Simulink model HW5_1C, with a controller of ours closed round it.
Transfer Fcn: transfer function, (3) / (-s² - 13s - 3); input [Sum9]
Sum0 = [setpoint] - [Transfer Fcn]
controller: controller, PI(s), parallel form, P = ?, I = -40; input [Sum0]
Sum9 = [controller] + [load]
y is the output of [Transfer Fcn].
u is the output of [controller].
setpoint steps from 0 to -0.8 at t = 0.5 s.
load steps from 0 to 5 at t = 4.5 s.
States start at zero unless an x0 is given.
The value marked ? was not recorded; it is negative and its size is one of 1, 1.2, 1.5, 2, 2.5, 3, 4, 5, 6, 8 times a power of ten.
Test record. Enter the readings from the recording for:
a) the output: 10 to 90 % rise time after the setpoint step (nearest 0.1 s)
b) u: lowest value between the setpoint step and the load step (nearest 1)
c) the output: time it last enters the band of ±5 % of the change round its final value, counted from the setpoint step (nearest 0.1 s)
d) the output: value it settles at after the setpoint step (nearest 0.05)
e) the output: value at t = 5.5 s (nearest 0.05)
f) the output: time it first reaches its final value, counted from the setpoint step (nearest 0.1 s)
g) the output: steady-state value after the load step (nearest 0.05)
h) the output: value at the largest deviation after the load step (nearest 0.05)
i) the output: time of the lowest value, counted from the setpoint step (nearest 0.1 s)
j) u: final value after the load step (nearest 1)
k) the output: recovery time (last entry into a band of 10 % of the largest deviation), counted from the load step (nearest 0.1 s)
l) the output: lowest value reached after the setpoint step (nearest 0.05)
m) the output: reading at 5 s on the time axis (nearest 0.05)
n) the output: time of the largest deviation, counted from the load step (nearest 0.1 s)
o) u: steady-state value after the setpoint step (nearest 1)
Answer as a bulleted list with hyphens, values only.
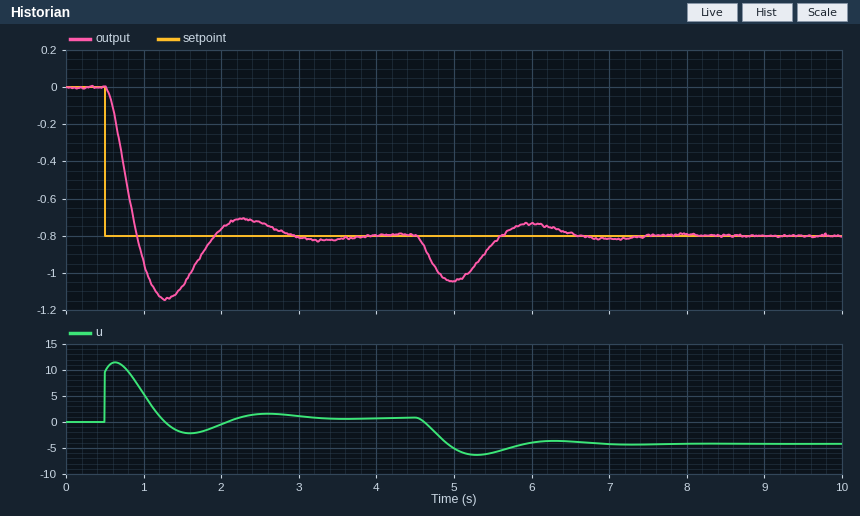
- 0.3 s
- -2
- 2.2 s
- -0.80
- -0.85
- 0.4 s
- -0.80
- -1.05
- 0.8 s
- -4
- 1.9 s
- -1.15
- -1.05
- 0.5 s
- 1
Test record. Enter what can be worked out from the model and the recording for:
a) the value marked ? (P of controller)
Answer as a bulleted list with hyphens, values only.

- -12
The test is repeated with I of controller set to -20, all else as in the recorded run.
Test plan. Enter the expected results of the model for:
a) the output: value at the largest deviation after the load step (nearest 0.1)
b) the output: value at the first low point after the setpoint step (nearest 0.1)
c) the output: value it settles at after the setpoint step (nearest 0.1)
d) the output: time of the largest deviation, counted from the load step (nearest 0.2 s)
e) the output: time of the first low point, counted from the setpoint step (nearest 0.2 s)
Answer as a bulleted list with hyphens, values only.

- -1.1
- -1.0
- -0.8
- 0.6 s
- 1.0 s
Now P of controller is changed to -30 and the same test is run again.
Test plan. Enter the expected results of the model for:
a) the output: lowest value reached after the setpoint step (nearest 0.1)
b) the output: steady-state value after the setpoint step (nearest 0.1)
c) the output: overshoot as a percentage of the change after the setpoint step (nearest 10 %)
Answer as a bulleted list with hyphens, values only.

- -1.0
- -0.8
- 20 %
